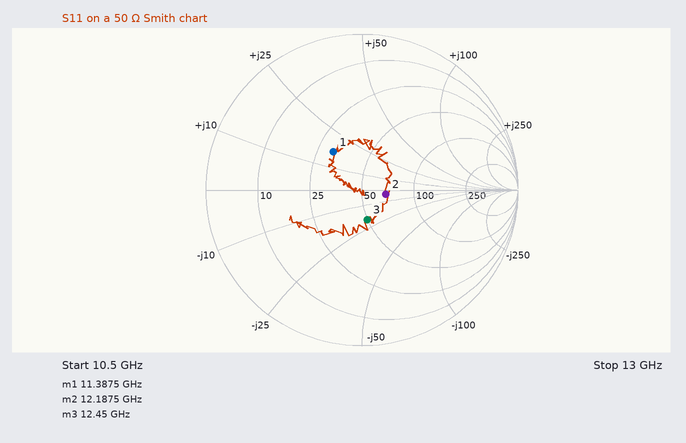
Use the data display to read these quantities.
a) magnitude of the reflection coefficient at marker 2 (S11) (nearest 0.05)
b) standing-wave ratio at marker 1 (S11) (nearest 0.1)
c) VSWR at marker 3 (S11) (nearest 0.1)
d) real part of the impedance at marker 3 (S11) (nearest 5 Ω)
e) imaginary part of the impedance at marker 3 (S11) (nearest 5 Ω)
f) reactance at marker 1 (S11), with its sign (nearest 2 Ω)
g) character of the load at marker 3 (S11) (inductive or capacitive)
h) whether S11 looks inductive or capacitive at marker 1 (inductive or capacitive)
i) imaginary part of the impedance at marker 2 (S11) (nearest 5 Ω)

0.15
1.9
1.5
50 Ω
-20 Ω
+16 Ω
capacitive
inductive
-5 Ω
